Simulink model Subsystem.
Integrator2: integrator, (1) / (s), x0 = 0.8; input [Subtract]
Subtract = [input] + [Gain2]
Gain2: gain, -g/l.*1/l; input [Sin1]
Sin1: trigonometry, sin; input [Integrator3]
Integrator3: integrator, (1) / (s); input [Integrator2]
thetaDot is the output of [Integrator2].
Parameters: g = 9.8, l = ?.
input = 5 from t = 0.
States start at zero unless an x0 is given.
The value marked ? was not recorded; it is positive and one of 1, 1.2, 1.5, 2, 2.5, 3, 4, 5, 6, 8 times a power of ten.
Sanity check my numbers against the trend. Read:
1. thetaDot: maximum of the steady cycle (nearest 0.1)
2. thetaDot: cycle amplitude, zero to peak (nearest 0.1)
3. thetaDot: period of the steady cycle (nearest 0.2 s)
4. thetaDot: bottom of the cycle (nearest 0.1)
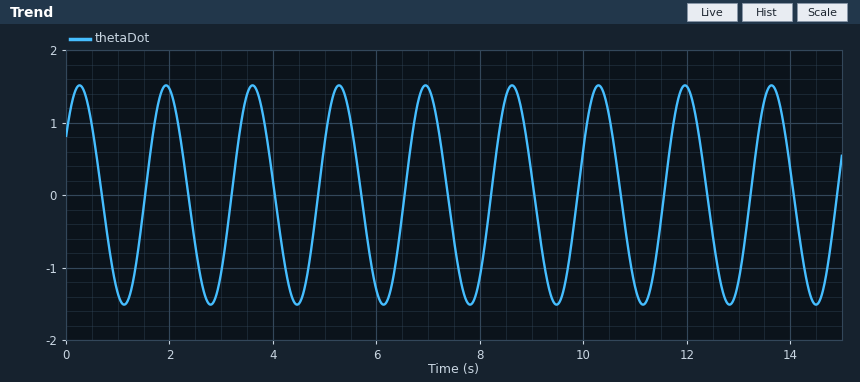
1.5
1.5
1.6 s
-1.5
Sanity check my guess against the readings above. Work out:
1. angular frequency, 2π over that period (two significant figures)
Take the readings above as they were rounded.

3.9 rad/s
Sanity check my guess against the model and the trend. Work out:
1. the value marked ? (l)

0.8
